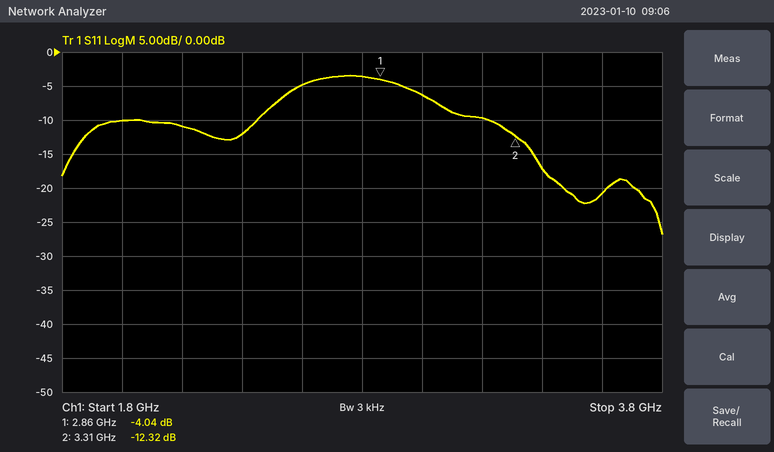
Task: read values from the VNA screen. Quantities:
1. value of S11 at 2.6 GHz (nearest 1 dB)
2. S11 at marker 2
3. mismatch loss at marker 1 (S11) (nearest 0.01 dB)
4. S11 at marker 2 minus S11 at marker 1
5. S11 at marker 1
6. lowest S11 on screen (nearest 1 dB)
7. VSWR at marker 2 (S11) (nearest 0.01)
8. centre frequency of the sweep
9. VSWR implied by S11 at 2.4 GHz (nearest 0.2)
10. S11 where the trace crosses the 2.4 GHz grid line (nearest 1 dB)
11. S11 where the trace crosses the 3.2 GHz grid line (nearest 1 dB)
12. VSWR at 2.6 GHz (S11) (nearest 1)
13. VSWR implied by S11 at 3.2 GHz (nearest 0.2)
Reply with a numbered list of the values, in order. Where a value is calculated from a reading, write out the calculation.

1. -5 dB
2. -12.32 dB
3. −10 log10(1 − 10^(-4.04/10)) ≈ 2.18 dB
4. -12.32 − (-4.04) = -8.28 dB
5. -4.04 dB
6. -27 dB
7. (1 + 0.2421)/(1 − 0.2421) ≈ 1.64
8. 2.8 GHz
9. |Γ| = 10^(-12/20) = 0.2512; VSWR = (1 + 0.2512)/(1 − 0.2512) ≈ 1.67, so 1.6 to the nearest 0.2
10. -12 dB
11. -10 dB
12. |Γ| = 10^(-5/20) = 0.5623; VSWR = (1 + 0.5623)/(1 − 0.5623) ≈ 4
13. |Γ| = 10^(-10/20) = 0.3162; VSWR = (1 + 0.3162)/(1 − 0.3162) ≈ 1.92, so 2.0 to the nearest 0.2
